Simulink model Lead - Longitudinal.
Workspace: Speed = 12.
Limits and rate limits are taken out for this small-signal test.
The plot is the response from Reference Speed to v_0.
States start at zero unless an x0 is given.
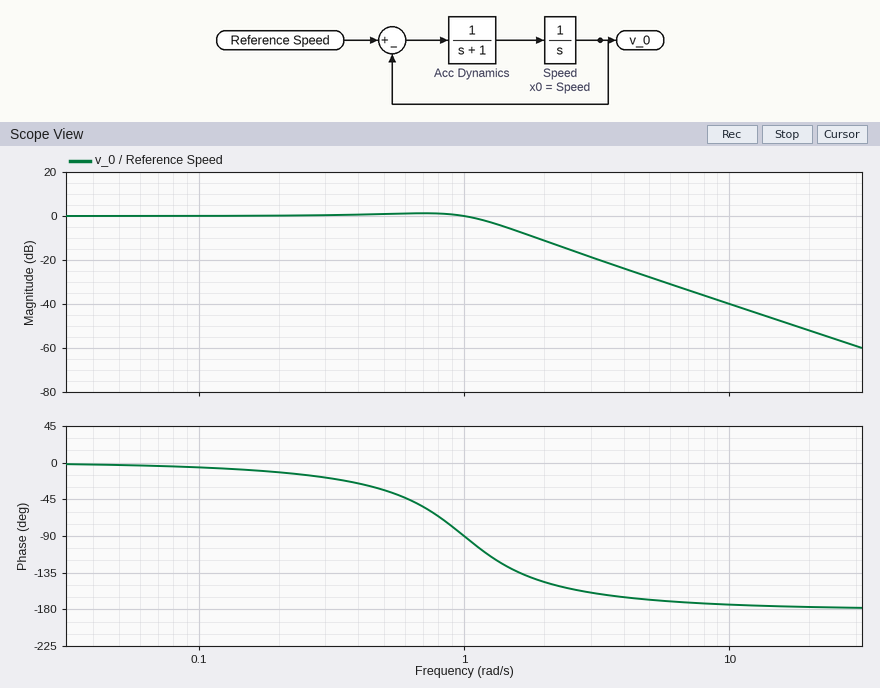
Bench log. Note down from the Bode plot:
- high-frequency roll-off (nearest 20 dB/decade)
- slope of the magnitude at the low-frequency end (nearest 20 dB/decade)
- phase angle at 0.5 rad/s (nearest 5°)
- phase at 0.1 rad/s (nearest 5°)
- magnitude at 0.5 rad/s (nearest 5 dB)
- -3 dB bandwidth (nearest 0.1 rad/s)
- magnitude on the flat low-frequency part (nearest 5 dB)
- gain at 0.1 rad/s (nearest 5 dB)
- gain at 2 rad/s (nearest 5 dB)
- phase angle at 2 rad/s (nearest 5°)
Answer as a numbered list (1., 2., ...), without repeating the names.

1. -40 dB/decade
2. 0 dB/decade
3. -35°
4. -5°
5. 0 dB
6. 1.3 rad/s
7. 0 dB
8. 0 dB
9. -10 dB
10. -145°
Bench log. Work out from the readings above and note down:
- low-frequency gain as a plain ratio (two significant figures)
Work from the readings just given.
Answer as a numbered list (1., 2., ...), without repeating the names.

1. 1.0
